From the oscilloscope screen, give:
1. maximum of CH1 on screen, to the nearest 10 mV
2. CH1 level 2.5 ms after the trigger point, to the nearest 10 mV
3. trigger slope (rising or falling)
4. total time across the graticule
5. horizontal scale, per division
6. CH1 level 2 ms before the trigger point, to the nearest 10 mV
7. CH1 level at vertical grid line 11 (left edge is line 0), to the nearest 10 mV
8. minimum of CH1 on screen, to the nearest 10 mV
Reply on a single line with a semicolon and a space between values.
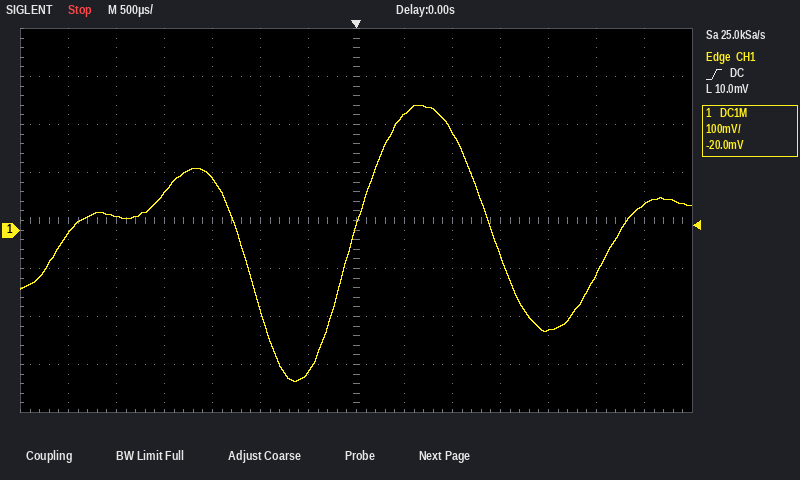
260 mV; -90 mV; rising; 7 ms; 500 µs; 80 mV; -210 mV; -320 mV
